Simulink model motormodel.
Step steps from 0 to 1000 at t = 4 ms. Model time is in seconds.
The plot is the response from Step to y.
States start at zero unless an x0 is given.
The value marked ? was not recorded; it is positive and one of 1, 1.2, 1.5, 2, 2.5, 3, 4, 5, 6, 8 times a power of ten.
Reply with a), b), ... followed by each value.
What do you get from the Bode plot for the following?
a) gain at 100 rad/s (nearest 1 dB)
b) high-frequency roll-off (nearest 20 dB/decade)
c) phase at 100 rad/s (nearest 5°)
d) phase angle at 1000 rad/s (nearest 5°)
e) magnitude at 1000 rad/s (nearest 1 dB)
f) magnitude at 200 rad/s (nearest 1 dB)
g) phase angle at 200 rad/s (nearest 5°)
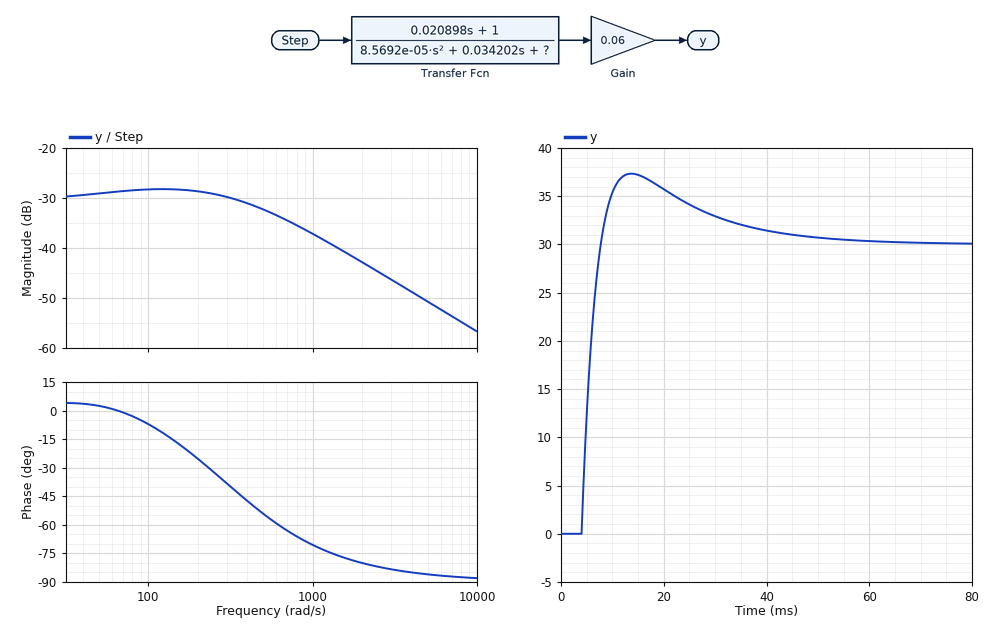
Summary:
a) -28 dB
b) -20 dB/decade
c) -5°
d) -70°
e) -37 dB
f) -29 dB
g) -25°
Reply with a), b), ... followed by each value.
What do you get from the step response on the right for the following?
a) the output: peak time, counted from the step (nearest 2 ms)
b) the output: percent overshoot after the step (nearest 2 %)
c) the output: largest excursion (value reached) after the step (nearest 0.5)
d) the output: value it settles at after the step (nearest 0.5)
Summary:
a) 10 ms
b) 24 %
c) 37.5
d) 30.0
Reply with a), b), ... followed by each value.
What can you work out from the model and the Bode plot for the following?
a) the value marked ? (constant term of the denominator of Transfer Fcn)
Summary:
a) 2
